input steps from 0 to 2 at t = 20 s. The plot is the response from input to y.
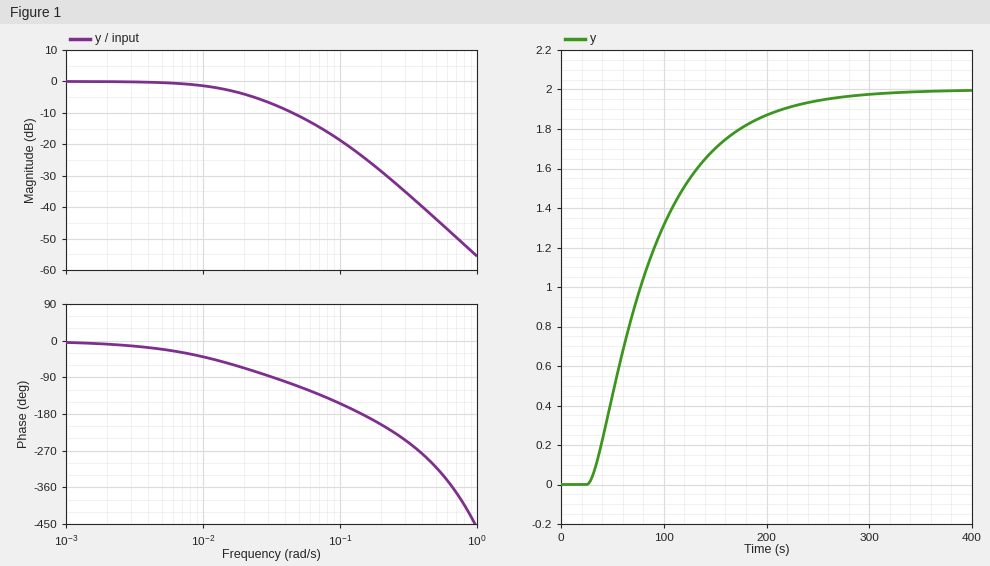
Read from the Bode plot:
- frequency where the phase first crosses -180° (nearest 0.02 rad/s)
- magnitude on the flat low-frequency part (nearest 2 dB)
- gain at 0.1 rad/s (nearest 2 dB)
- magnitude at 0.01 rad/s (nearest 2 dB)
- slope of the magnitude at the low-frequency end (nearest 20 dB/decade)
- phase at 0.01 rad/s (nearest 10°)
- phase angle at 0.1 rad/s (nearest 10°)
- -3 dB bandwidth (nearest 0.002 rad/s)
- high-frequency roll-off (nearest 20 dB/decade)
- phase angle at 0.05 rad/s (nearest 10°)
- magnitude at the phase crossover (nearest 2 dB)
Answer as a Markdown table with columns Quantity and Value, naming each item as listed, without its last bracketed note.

| Quantity | Value |
|---|---|
| frequency where the phase first crosses -180° | 0.14 rad/s |
| magnitude on the flat low-frequency part | 0 dB |
| gain at 0.1 rad/s | -18 dB |
| magnitude at 0.01 rad/s | -2 dB |
| slope of the magnitude at the low-frequency end | 0 dB/decade |
| phase at 0.01 rad/s | -40° |
| phase angle at 0.1 rad/s | -150° |
| -3 dB bandwidth | 0.016 rad/s |
| high-frequency roll-off | -40 dB/decade |
| phase angle at 0.05 rad/s | -110° |
| magnitude at the phase crossover | -24 dB |
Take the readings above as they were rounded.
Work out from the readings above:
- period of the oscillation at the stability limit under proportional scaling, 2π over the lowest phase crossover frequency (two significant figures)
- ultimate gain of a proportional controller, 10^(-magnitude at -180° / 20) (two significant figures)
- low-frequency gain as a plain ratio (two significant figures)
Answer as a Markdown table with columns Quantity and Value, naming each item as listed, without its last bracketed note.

| Quantity | Value |
|---|---|
| period of the oscillation at the stability limit under proportional scaling, 2π over the lowest phase crossover frequency | 45 s |
| ultimate gain of a proportional controller, 10^(-magnitude at -180° / 20) | 16 |
| low-frequency gain as a plain ratio | 1.0 |
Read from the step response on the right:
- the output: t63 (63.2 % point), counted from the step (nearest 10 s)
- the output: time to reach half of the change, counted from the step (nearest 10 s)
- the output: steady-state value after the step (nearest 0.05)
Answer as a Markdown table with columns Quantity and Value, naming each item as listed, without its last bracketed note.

| Quantity | Value |
|---|---|
| the output: t63 (63.2 % point), counted from the step | 80 s |
| the output: time to reach half of the change, counted from the step | 60 s |
| the output: steady-state value after the step | 2.00 |
